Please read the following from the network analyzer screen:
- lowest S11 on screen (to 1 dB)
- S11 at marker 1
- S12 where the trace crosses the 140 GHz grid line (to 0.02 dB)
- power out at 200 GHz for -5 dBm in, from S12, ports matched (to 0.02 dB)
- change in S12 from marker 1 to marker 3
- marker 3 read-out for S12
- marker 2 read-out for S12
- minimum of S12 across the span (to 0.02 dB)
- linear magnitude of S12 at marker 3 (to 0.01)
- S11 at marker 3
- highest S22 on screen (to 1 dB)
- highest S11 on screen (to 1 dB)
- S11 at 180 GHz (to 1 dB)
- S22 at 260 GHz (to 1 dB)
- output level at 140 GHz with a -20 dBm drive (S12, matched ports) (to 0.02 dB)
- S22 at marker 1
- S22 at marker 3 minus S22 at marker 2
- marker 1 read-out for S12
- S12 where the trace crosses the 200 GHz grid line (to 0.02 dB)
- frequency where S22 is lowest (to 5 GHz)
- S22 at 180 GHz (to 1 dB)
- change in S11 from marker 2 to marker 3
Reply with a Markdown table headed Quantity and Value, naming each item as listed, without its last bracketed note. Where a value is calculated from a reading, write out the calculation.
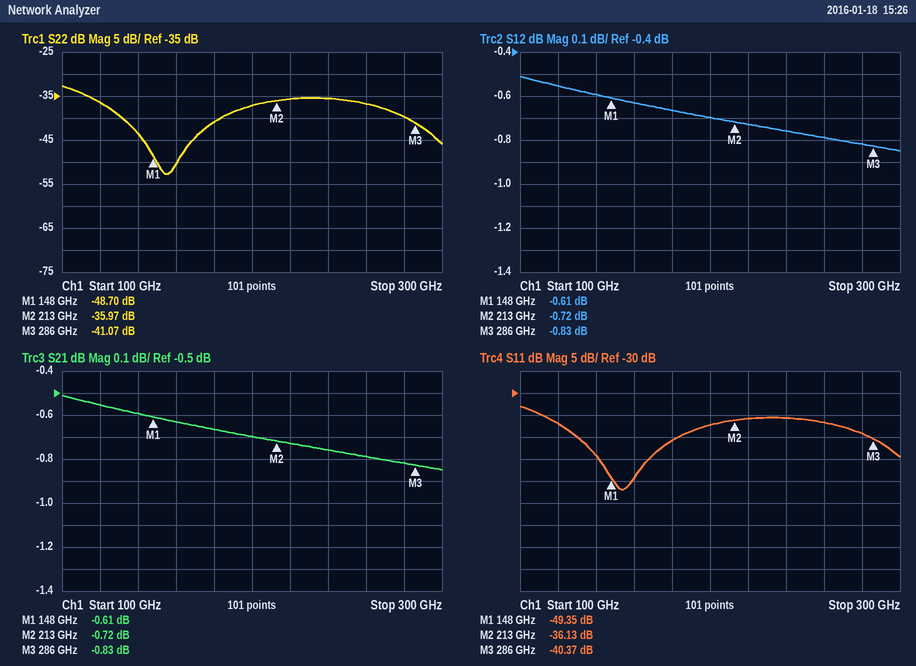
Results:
| Quantity | Value |
|---|---|
| lowest S11 on screen | -52 dB |
| S11 at marker 1 | -49.35 dB |
| S12 where the trace crosses the 140 GHz grid line | -0.60 dB |
| power out at 200 GHz for -5 dBm in, from S12, ports matched | -5 dBm + (-0.70 dB) = -5.70 dBm |
| change in S12 from marker 1 to marker 3 | -0.83 − (-0.61) = -0.22 dB |
| marker 3 read-out for S12 | -0.83 dB |
| marker 2 read-out for S12 | -0.72 dB |
| minimum of S12 across the span | -0.84 dB |
| linear magnitude of S12 at marker 3 | 10^(-0.83/20) ≈ 0.91 |
| S11 at marker 3 | -40.37 dB |
| highest S22 on screen | -33 dB |
| highest S11 on screen | -33 dB |
| S11 at 180 GHz | -41 dB |
| S22 at 260 GHz | -37 dB |
| output level at 140 GHz with a -20 dBm drive (S12, matched ports) | -20 dBm + (-0.60 dB) = -20.60 dBm |
| S22 at marker 1 | -48.70 dB |
| S22 at marker 3 minus S22 at marker 2 | -41.07 − (-35.97) = -5.10 dB |
| marker 1 read-out for S12 | -0.61 dB |
| S12 where the trace crosses the 200 GHz grid line | -0.70 dB |
| frequency where S22 is lowest | 155 GHz |
| S22 at 180 GHz | -41 dB |
| change in S11 from marker 2 to marker 3 | -40.37 − (-36.13) = -4.24 dB |
